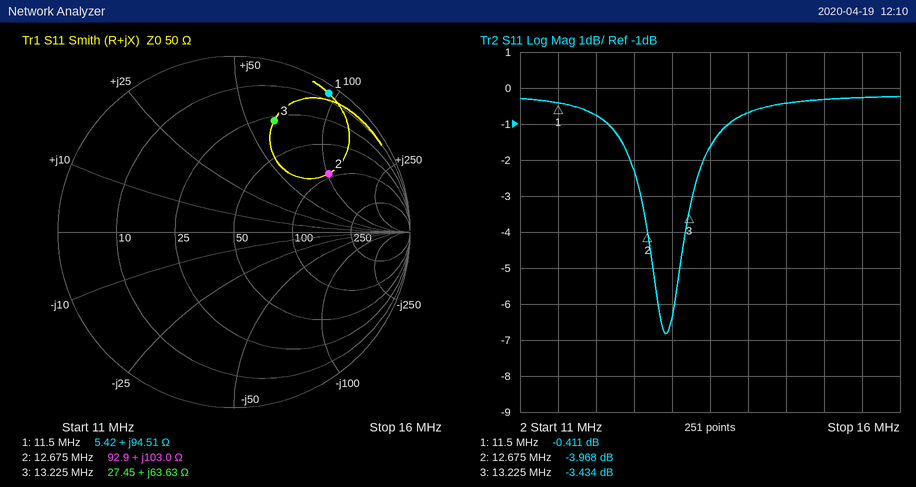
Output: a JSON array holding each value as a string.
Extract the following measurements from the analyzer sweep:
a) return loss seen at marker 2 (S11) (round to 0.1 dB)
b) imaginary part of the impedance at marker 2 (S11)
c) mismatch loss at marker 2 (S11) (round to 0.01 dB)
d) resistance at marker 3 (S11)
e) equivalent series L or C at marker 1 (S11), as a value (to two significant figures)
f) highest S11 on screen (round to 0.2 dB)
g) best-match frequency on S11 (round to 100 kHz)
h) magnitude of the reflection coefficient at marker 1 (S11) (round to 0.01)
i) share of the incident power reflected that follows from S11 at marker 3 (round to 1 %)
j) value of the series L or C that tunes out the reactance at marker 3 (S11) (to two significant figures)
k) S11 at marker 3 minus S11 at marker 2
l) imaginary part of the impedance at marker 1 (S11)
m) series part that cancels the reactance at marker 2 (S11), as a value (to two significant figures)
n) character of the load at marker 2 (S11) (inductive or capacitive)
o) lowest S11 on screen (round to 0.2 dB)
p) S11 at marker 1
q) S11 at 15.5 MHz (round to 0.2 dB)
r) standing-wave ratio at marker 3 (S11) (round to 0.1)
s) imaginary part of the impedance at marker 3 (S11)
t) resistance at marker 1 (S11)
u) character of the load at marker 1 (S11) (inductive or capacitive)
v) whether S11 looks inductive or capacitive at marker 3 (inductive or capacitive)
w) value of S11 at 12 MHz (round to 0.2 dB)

["4.0 dB", "+103.0 Ω", "2.23 dB", "27.45 Ω", "1.3 µH", "-0.2 dB", "12.9 MHz", "0.95", "45 %", "190 pF", "0.534 dB", "+94.51 Ω", "120 pF", "inductive", "-6.8 dB", "-0.411 dB", "-0.2 dB", "5.1", "+63.63 Ω", "5.42 Ω", "inductive", "inductive", "-0.8 dB"]
